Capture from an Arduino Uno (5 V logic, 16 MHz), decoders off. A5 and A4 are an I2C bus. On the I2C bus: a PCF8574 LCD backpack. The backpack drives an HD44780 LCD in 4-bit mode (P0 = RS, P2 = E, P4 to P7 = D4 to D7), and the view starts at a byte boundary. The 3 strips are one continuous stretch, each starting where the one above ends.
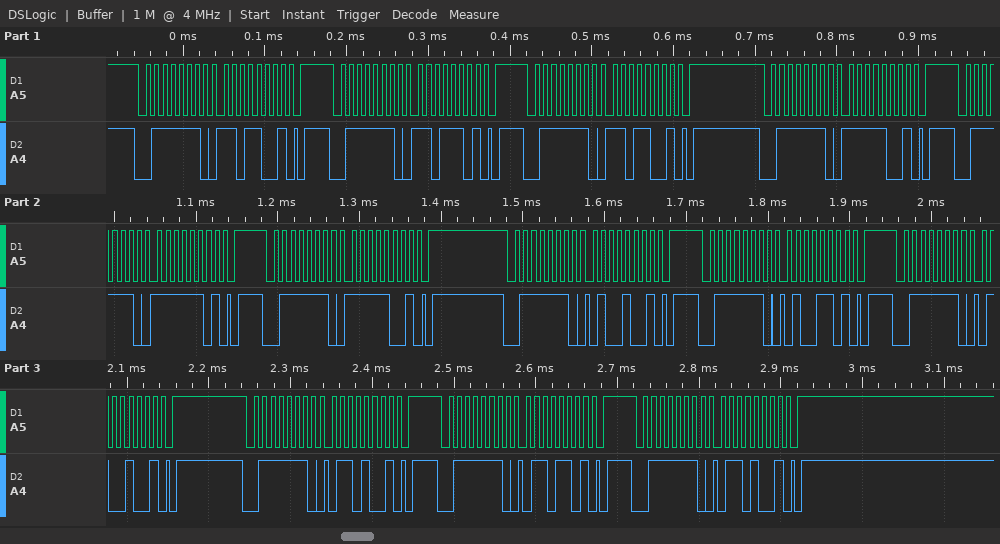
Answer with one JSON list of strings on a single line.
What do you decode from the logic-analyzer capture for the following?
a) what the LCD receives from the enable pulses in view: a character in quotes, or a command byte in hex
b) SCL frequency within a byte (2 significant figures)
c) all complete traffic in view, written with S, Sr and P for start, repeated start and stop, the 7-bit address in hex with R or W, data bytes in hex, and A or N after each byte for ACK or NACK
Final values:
["data 0xDF 'F'", "100 kHz", "S 3FW A D9 A P S 3FW A DD A P S 3FW A D9 A P S 3FW A F9 A P S 3FW A FD A P S 3FW A F9 A P S 3FW A 49 A P S 3FW A 4D A P S 3FW A 49 A P S 3FW A 69 A P S 3FW A 6D A P S 3FW A 69 A P"]
